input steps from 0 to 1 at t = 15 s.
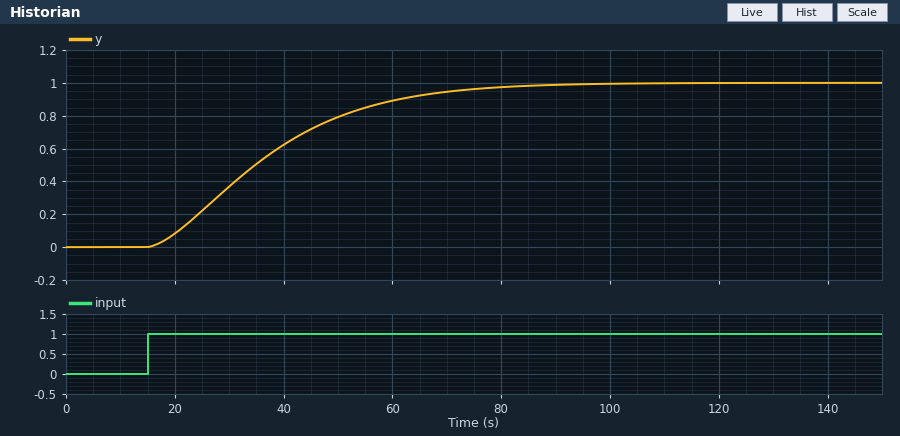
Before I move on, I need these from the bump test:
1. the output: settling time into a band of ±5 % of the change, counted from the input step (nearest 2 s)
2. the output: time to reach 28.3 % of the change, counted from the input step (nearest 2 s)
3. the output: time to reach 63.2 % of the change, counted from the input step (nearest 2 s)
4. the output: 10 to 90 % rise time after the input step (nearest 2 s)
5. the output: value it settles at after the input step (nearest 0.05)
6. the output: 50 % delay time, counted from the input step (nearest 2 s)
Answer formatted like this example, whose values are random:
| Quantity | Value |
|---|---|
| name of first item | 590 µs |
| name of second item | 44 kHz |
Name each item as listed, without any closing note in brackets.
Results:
| Quantity | Value |
|---|---|
| the output: settling time into a band of ±5 % of the change, counted from the input step | 56 s |
| the output: time to reach 28.3 % of the change, counted from the input step | 12 s |
| the output: time to reach 63.2 % of the change, counted from the input step | 26 s |
| the output: 10 to 90 % rise time after the input step | 40 s |
| the output: value it settles at after the input step | 1.00 |
| the output: 50 % delay time, counted from the input step | 20 s |
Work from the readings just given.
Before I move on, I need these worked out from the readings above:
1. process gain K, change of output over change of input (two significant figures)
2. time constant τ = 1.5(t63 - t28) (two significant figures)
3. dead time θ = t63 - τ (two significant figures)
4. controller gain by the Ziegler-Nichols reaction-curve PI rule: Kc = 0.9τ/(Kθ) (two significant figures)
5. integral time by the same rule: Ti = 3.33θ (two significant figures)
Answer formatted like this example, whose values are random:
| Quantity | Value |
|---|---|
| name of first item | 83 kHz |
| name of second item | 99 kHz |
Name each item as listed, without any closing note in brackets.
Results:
| Quantity | Value |
|---|---|
| process gain K, change of output over change of input | 1.0 |
| time constant τ = 1.5(t63 - t28) | 21 s |
| dead time θ = t63 - τ | 5.0 s |
| controller gain by the Ziegler-Nichols reaction-curve PI rule: Kc = 0.9τ/(Kθ) | 3.8 |
| integral time by the same rule: Ti = 3.33θ | 17 s |
